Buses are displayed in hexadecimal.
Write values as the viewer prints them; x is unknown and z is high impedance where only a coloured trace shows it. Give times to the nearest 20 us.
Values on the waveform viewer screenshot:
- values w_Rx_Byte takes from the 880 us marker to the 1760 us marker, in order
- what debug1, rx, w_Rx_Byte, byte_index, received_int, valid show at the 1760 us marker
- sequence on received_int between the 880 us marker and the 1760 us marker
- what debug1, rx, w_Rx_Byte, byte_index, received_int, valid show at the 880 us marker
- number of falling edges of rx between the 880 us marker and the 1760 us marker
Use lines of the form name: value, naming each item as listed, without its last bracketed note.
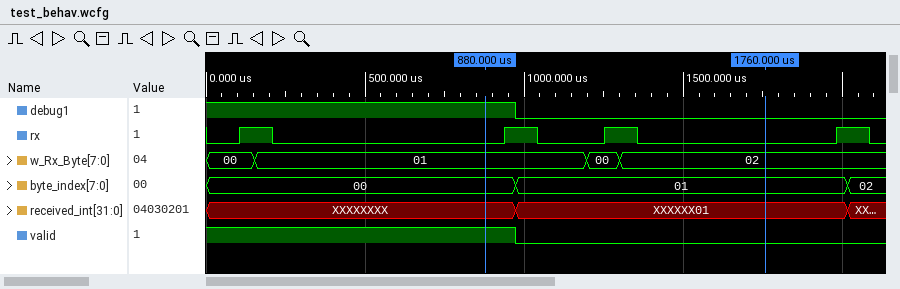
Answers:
values w_Rx_Byte takes from the 880 us marker to the 1760 us marker, in order: 01, 00, 02
what debug1, rx, w_Rx_Byte, byte_index, received_int, valid show at the 1760 us marker: debug1=0, rx=0, w_Rx_Byte=02, byte_index=01, received_int=XXXXXX01, valid=0
sequence on received_int between the 880 us marker and the 1760 us marker: XXXXXXXX, XXXXXX01
what debug1, rx, w_Rx_Byte, byte_index, received_int, valid show at the 880 us marker: debug1=1, rx=0, w_Rx_Byte=01, byte_index=00, received_int=XXXXXXXX, valid=1
number of falling edges of rx between the 880 us marker and the 1760 us marker: 2
